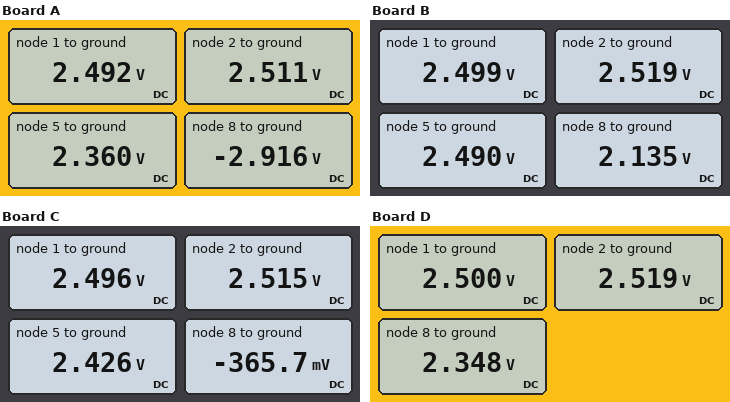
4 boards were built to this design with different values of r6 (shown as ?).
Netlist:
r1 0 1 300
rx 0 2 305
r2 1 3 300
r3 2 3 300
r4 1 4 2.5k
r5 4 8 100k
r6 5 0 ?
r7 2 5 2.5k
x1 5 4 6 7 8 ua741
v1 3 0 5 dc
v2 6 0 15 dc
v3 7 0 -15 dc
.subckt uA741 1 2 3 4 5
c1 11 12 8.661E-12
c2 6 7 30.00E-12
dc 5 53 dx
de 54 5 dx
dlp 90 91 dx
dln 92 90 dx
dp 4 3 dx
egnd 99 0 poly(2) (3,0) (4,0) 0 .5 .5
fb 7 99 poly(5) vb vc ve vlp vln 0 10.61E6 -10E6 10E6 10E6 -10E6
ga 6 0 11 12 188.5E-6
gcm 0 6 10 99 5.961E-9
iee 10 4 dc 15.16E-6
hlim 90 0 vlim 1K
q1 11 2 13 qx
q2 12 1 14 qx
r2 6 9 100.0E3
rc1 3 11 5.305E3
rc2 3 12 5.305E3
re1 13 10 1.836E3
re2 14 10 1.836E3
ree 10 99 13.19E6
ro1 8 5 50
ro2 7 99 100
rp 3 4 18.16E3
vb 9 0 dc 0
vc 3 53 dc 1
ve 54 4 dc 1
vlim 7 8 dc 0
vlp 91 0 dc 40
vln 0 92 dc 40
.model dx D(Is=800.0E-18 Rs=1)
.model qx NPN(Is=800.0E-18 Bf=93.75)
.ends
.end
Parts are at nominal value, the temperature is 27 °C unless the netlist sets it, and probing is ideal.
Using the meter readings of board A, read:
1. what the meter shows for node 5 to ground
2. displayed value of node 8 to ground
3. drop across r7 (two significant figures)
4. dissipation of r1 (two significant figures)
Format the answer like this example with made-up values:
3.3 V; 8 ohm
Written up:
2.360 V; -2.916 V; 150 mV; 21 mW
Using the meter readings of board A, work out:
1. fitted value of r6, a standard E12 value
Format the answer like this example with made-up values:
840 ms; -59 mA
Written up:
39 kΩ
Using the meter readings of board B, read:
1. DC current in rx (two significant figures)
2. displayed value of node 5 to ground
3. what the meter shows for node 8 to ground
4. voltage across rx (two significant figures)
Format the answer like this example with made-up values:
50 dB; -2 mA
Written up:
8.3 mA; 2.490 V; 2.135 V; 2.5 V
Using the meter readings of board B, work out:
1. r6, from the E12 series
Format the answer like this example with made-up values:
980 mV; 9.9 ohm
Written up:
220 kΩ
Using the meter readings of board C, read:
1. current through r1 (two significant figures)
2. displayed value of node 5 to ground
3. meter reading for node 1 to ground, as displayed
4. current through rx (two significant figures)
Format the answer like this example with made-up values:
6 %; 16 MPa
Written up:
8.3 mA; 2.426 V; 2.496 V; 8.2 mA
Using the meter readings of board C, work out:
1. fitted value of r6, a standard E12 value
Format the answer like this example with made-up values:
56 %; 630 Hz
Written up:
68 kΩ
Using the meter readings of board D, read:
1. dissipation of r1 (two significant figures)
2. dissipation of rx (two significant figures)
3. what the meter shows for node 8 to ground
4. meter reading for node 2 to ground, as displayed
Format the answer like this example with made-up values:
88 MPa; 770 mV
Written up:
21 mW; 21 mW; 2.348 V; 2.519 V
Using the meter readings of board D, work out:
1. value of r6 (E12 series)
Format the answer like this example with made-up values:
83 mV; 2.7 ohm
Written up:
270 kΩ
